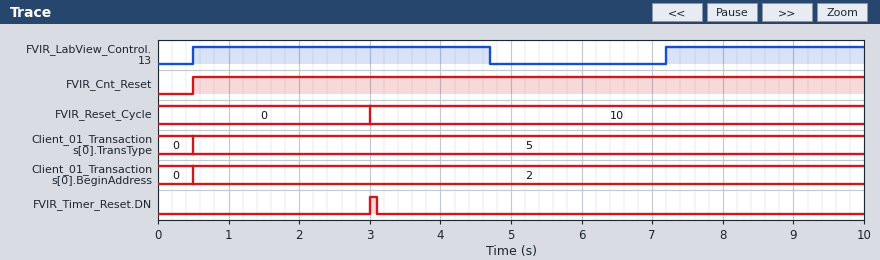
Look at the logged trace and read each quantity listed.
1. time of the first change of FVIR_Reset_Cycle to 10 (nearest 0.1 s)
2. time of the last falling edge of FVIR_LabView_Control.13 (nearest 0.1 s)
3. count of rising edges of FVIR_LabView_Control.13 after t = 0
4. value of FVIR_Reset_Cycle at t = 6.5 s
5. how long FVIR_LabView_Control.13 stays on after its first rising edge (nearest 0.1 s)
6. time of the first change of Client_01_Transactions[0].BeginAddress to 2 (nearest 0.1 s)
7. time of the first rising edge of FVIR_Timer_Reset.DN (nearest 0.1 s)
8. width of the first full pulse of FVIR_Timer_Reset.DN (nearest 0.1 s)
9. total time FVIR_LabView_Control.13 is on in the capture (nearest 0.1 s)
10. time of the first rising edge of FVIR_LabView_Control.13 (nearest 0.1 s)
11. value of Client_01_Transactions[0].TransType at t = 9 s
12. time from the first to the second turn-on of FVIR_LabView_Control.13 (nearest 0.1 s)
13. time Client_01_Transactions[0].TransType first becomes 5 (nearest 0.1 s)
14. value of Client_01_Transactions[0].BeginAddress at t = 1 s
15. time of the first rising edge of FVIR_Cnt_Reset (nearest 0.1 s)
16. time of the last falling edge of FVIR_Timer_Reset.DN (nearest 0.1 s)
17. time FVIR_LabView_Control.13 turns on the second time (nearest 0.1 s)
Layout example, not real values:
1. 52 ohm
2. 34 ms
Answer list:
1. 3.0 s
2. 4.7 s
3. 2
4. 10
5. 4.2 s
6. 0.5 s
7. 3.0 s
8. 0.1 s
9. 7.0 s
10. 0.5 s
11. 5
12. 6.7 s
13. 0.5 s
14. 2
15. 0.5 s
16. 3.1 s
17. 7.2 s
